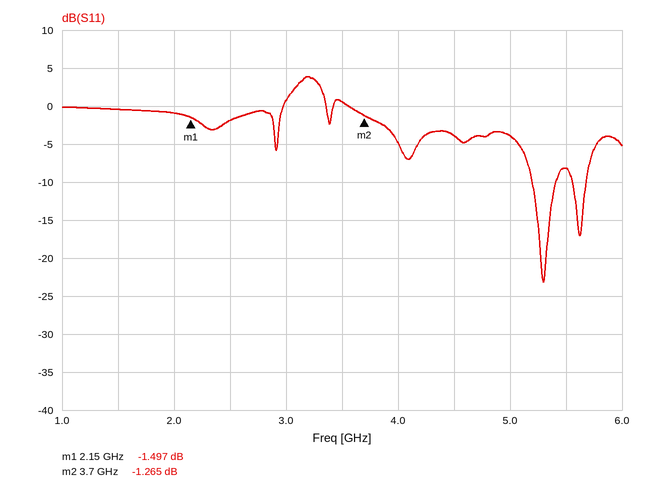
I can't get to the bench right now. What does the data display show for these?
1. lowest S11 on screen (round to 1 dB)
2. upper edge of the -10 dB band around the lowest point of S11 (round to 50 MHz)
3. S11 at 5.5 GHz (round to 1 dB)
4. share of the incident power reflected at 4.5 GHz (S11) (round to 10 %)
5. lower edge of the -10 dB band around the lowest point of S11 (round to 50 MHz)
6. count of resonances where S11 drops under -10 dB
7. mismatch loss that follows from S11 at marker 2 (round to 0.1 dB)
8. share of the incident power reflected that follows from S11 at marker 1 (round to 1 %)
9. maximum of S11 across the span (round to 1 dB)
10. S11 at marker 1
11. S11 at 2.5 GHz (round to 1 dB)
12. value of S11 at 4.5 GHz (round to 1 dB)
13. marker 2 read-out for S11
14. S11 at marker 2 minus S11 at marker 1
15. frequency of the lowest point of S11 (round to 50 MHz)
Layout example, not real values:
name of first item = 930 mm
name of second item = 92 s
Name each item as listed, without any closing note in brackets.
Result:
lowest S11 on screen = -23 dB
upper edge of the -10 dB band around the lowest point of S11 = 5.40 GHz
S11 at 5.5 GHz = -8 dB
share of the incident power reflected at 4.5 GHz (S11) = 40 %
lower edge of the -10 dB band around the lowest point of S11 = 5.20 GHz
count of resonances where S11 drops under -10 dB = 2
mismatch loss that follows from S11 at marker 2 = 6.0 dB
share of the incident power reflected that follows from S11 at marker 1 = 71 %
maximum of S11 across the span = 4 dB
S11 at marker 1 = -1.497 dB
S11 at 2.5 GHz = -2 dB
value of S11 at 4.5 GHz = -4 dB
marker 2 read-out for S11 = -1.265 dB
S11 at marker 2 minus S11 at marker 1 = 0.232 dB
frequency of the lowest point of S11 = 5.30 GHz
